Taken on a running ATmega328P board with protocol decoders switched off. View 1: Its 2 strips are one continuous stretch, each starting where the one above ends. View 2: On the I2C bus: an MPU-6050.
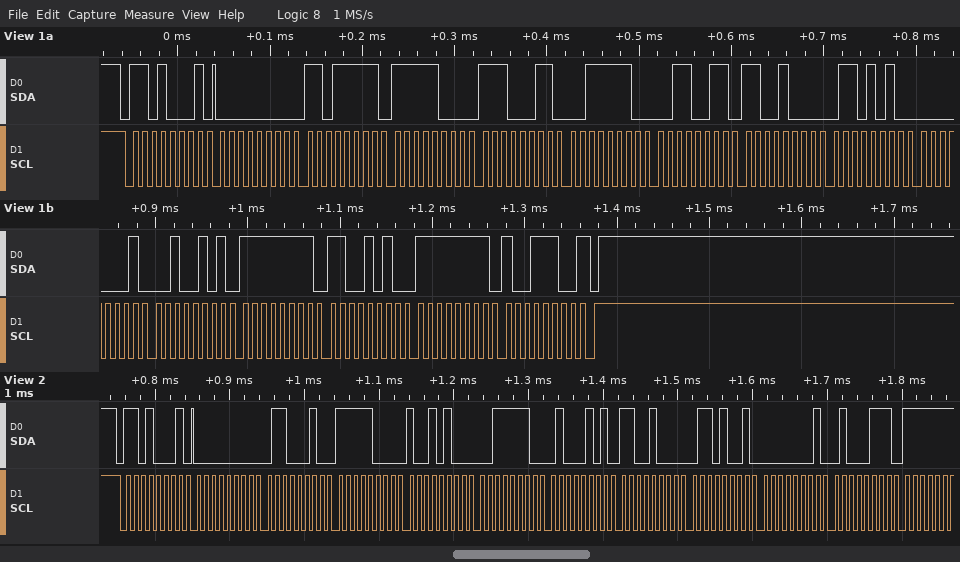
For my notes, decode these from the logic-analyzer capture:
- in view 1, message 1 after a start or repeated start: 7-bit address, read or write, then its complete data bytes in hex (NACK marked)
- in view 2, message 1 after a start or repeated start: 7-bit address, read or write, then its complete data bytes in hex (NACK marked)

0x68 read: 00 DF F8 E3 3E 33 C8 6A 01 25 FF CA FF 9C NACK
0x68 read: 00 62 F8 94 3E 45 C8 69 01 47
